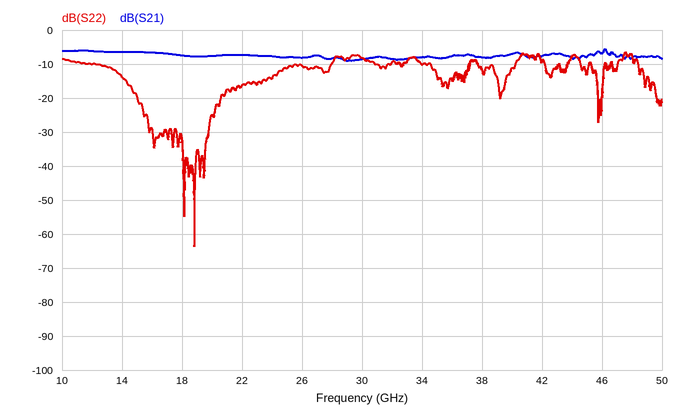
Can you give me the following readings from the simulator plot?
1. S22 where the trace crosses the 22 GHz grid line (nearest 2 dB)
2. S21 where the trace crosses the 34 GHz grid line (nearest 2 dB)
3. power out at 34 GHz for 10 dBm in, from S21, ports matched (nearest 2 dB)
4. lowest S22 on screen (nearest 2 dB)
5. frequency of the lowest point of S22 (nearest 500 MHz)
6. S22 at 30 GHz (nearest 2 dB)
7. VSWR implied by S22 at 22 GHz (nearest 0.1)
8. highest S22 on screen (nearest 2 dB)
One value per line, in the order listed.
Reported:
-16 dB
-8 dB
2 dBm
-64 dB
19.0 GHz
-8 dB
1.4
-6 dB
